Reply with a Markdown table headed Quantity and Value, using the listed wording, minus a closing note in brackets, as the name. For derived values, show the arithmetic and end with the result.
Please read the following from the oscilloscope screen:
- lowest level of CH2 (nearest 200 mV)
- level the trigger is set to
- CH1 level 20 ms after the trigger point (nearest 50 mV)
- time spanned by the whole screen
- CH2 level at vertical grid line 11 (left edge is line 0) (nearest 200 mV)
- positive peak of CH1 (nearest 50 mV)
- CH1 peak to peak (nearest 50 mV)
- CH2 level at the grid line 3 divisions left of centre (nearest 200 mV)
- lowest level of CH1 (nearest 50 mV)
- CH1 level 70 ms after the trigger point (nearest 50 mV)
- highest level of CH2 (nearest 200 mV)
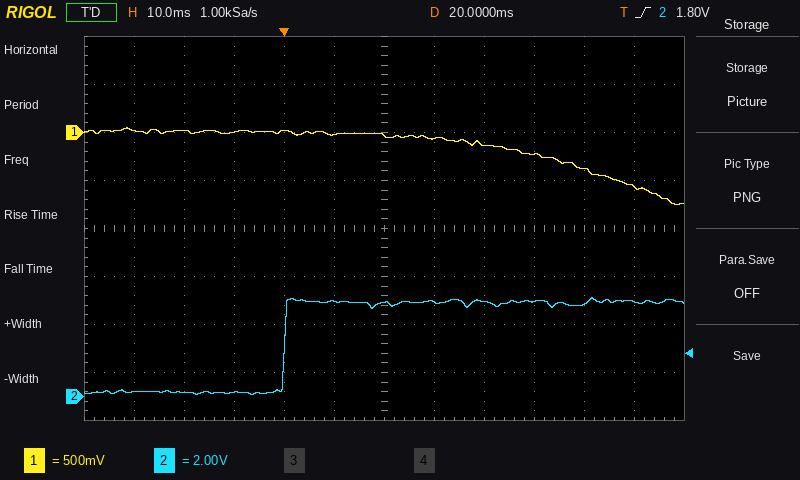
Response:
| Quantity | Value |
|---|---|
| lowest level of CH2 | 0.0 V |
| level the trigger is set to | 1.80 V |
| CH1 level 20 ms after the trigger point | -50 mV |
| time spanned by the whole screen | 120 ms |
| CH2 level at vertical grid line 11 (left edge is line 0) | 4.0 V |
| positive peak of CH1 | 50 mV |
| CH1 peak to peak | 50 mV − (-750 mV) = 800 mV |
| CH2 level at the grid line 3 divisions left of centre | 200 mV |
| lowest level of CH1 | -750 mV |
| CH1 level 70 ms after the trigger point | -550 mV |
| highest level of CH2 | 4.2 V |
